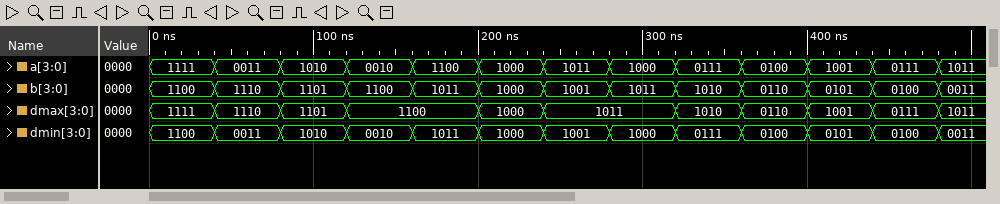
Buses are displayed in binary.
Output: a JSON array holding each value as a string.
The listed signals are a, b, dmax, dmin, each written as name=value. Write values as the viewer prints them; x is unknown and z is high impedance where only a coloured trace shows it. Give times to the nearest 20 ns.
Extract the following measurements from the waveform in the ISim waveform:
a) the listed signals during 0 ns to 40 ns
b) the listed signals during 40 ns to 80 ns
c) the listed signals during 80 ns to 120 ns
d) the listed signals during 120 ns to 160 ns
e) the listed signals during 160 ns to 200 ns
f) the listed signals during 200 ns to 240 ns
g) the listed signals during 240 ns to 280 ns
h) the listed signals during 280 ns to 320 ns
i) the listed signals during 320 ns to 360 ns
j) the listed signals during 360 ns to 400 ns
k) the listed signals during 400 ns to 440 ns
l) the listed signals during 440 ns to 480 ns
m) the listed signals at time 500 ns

["a=1111, b=1100, dmax=1111, dmin=1100", "a=0011, b=1110, dmax=1110, dmin=0011", "a=1010, b=1101, dmax=1101, dmin=1010", "a=0010, b=1100, dmax=1100, dmin=0010", "a=1100, b=1011, dmax=1100, dmin=1011", "a=1000, b=1000, dmax=1000, dmin=1000", "a=1011, b=1001, dmax=1011, dmin=1001", "a=1000, b=1011, dmax=1011, dmin=1000", "a=0111, b=1010, dmax=1010, dmin=0111", "a=0100, b=0110, dmax=0110, dmin=0100", "a=1001, b=0101, dmax=1001, dmin=0101", "a=0111, b=0100, dmax=0111, dmin=0100", "a=1011, b=0011, dmax=1011, dmin=0011"]
